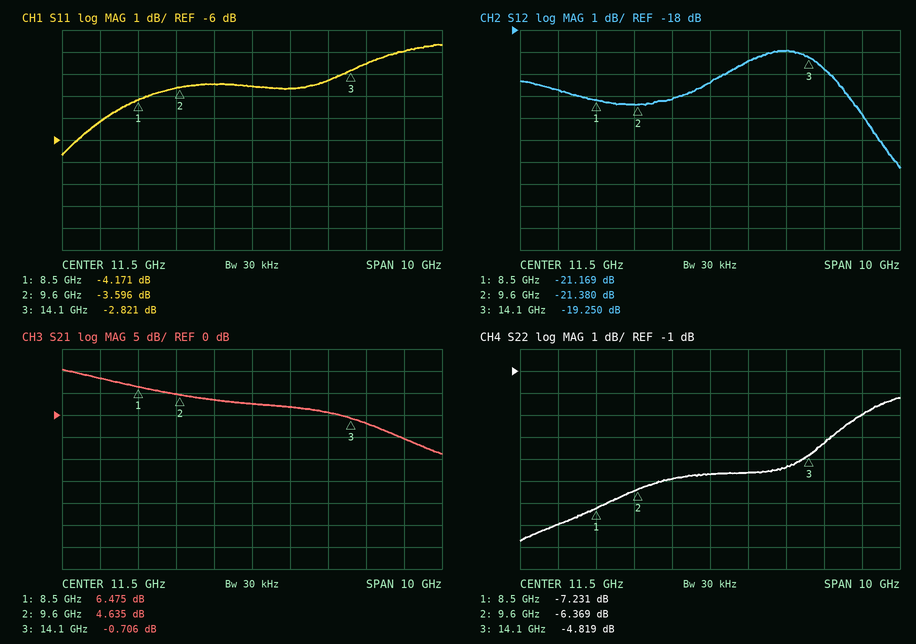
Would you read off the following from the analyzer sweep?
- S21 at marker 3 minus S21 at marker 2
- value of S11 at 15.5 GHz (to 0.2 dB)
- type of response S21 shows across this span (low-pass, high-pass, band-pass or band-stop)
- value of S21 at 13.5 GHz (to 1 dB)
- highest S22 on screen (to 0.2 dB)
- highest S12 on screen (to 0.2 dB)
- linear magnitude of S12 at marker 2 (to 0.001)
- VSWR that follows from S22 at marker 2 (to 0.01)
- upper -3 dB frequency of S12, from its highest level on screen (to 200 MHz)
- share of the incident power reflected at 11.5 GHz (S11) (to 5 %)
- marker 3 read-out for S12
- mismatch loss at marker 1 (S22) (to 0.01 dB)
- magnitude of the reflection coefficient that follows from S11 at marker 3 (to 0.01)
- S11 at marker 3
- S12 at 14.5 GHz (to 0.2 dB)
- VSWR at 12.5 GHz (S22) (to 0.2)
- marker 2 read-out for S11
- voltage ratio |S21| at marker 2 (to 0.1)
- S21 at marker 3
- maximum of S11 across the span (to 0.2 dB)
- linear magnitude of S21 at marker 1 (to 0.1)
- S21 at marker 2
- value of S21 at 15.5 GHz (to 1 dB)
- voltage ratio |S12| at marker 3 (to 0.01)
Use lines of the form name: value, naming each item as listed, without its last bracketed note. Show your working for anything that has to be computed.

S21 at marker 3 minus S21 at marker 2: -0.706 − (4.635) = -5.341 dB
value of S11 at 15.5 GHz: -2.0 dB
type of response S21 shows across this span: low-pass
value of S21 at 13.5 GHz: 1 dB
highest S22 on screen: -2.2 dB
highest S12 on screen: -19.0 dB
linear magnitude of S12 at marker 2: 10^(-21.38/20) ≈ 0.085
VSWR that follows from S22 at marker 2: (1 + 0.4803)/(1 − 0.4803) ≈ 2.85
upper -3 dB frequency of S12, from its highest level on screen: 15.6 GHz
share of the incident power reflected at 11.5 GHz (S11): 10^(-3.6/10) ≈ 43.7 %, so 45 % to the nearest 5 %
marker 3 read-out for S12: -19.250 dB
mismatch loss at marker 1 (S22): −10 log10(1 − 10^(-7.231/10)) ≈ 0.91 dB
magnitude of the reflection coefficient that follows from S11 at marker 3: 10^(-2.821/20) ≈ 0.72
S11 at marker 3: -2.821 dB
S12 at 14.5 GHz: -19.8 dB
VSWR at 12.5 GHz (S22): |Γ| = 10^(-5.6/20) = 0.5248; VSWR = (1 + 0.5248)/(1 − 0.5248) ≈ 3.2
marker 2 read-out for S11: -3.596 dB
voltage ratio |S21| at marker 2: 10^(4.635/20) ≈ 1.7
S21 at marker 3: -0.706 dB
maximum of S11 across the span: -1.6 dB
linear magnitude of S21 at marker 1: 10^(6.475/20) ≈ 2.1
S21 at marker 2: 4.635 dB
value of S21 at 15.5 GHz: -5 dB
voltage ratio |S12| at marker 3: 10^(-19.25/20) ≈ 0.11
